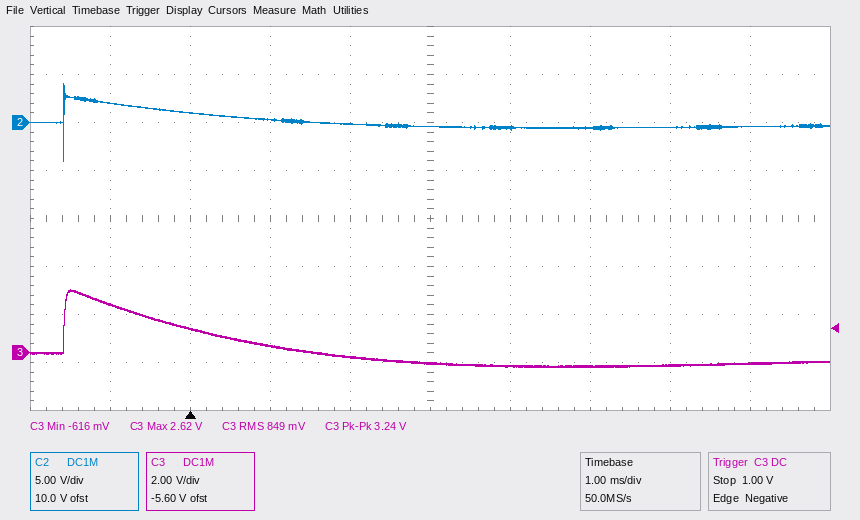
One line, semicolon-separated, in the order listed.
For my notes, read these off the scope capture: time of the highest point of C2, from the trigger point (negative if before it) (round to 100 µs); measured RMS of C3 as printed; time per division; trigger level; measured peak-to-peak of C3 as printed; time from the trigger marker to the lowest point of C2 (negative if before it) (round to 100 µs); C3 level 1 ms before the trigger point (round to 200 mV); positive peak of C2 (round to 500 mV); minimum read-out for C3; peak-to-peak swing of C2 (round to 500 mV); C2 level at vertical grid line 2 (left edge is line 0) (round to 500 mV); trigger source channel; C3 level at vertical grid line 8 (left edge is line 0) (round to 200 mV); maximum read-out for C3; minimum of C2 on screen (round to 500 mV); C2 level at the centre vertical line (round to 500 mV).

-1.6 ms; 849 mV; 1 ms; 1.00 V; 3.24 V; -1.6 ms; 2.0 V; 4.0 V; -616 mV; 8.0 V; 1.0 V; C3; -600 mV; 2.62 V; -4.0 V; -500 mV
